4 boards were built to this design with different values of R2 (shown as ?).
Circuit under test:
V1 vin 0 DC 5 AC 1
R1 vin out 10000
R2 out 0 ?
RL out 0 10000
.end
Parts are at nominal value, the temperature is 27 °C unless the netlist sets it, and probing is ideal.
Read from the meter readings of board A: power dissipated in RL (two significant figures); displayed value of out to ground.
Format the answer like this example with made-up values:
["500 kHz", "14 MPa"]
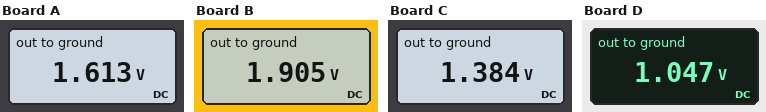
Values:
["260 µW", "1.613 V"]
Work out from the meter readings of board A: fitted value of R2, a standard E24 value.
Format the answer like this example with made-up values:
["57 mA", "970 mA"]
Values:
["9.1 kΩ"]
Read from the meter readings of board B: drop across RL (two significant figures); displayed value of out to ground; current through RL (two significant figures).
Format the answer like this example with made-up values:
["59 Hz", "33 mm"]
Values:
["1.9 V", "1.905 V", "190 µA"]
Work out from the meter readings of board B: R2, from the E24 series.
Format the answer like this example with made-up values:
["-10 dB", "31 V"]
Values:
["16 kΩ"]
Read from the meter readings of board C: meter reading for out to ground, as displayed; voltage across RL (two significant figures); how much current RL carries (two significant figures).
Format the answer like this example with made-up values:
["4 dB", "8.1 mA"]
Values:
["1.384 V", "1.4 V", "140 µA"]
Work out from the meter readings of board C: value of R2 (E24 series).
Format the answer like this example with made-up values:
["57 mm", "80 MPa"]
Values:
["6.2 kΩ"]
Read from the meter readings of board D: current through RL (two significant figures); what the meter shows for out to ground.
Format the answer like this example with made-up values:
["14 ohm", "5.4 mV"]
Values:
["100 µA", "1.047 V"]
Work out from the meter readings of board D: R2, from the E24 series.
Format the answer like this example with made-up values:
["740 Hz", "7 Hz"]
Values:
["3.6 kΩ"]
